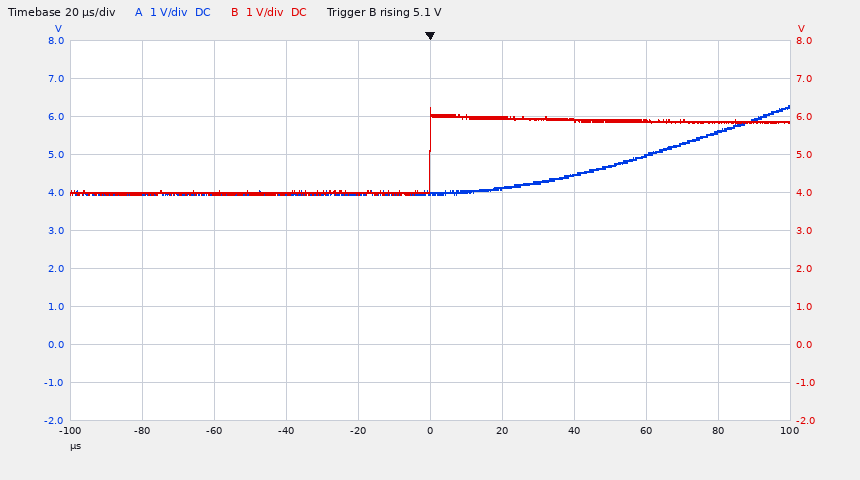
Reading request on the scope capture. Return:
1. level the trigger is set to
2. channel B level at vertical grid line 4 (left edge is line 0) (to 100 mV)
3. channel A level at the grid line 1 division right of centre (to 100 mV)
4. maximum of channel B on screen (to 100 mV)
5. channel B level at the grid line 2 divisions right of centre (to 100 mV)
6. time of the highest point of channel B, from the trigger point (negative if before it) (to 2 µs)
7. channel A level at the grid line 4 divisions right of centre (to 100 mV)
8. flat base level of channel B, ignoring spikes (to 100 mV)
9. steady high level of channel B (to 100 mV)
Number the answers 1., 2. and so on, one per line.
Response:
1. 5.1 V
2. 4.0 V
3. 4.1 V
4. 6.2 V
5. 5.9 V
6. 0 µs
7. 5.6 V
8. 4.0 V
9. 5.9 V
